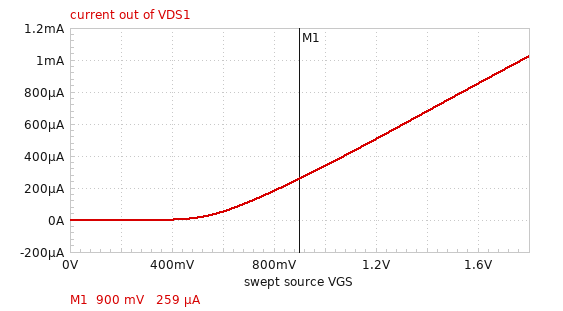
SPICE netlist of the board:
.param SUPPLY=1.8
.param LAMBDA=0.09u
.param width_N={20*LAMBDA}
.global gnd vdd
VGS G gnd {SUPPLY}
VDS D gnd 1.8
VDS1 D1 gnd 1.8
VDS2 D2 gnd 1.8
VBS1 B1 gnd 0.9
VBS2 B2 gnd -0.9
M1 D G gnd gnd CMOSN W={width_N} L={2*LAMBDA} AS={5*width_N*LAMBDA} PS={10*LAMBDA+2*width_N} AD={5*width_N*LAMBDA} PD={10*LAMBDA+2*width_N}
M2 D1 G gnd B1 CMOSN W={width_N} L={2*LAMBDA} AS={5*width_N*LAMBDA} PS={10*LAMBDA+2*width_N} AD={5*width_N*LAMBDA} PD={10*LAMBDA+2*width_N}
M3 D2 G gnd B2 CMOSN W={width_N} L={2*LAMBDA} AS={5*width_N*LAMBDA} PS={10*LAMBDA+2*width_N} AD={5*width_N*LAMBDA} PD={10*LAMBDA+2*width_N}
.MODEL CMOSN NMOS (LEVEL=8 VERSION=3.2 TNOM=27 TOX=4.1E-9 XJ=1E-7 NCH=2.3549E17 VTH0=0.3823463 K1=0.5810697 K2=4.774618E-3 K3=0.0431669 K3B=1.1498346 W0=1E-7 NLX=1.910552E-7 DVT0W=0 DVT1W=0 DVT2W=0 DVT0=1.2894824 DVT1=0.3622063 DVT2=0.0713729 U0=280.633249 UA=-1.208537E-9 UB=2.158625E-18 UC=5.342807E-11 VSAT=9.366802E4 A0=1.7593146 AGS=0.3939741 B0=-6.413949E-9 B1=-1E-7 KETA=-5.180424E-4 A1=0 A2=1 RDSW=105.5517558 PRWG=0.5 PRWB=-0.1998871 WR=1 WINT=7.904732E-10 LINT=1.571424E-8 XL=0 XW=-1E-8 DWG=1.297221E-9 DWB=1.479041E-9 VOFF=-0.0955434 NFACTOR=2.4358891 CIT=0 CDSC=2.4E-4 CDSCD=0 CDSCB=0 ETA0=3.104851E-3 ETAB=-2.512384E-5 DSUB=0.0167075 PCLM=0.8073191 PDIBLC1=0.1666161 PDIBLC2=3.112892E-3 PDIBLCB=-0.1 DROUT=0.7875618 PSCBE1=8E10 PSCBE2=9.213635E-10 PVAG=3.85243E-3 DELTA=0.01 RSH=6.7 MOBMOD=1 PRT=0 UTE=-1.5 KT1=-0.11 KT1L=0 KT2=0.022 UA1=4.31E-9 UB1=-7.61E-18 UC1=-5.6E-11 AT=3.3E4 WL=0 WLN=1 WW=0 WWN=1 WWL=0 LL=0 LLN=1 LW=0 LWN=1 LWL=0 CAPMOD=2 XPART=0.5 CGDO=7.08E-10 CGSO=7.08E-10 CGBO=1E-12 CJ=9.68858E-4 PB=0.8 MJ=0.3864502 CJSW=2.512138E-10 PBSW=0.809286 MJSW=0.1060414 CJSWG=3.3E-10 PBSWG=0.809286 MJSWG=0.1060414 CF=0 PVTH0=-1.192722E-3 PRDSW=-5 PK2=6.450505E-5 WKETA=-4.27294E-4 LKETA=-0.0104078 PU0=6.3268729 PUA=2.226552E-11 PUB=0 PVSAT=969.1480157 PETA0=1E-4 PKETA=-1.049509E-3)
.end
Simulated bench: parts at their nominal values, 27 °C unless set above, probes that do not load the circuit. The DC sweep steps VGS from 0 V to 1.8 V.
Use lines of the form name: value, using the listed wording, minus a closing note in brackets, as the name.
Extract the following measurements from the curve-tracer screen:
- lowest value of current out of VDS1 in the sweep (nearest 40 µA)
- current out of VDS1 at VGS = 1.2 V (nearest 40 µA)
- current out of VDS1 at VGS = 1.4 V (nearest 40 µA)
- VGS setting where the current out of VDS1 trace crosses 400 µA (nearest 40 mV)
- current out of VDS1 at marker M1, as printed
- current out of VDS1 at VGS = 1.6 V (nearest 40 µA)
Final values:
lowest value of current out of VDS1 in the sweep: 0 A
current out of VDS1 at VGS = 1.2 V: 520 µA
current out of VDS1 at VGS = 1.4 V: 680 µA
VGS setting where the current out of VDS1 trace crosses 400 µA: 1.08 V
current out of VDS1 at marker M1, as printed: 259 µA
current out of VDS1 at VGS = 1.6 V: 840 µA
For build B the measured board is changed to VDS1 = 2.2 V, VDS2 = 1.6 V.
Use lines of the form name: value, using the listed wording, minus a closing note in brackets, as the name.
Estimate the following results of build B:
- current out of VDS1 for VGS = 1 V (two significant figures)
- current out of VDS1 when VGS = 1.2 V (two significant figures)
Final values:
current out of VDS1 for VGS = 1 V: 350 µA
current out of VDS1 when VGS = 1.2 V: 520 µA
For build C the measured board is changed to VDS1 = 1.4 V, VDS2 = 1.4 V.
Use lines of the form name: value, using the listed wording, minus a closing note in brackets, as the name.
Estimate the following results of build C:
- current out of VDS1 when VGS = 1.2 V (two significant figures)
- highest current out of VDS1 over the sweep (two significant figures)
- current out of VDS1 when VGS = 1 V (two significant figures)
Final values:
current out of VDS1 when VGS = 1.2 V: 490 µA
highest current out of VDS1 over the sweep: 1.0 mA
current out of VDS1 when VGS = 1 V: 330 µA
